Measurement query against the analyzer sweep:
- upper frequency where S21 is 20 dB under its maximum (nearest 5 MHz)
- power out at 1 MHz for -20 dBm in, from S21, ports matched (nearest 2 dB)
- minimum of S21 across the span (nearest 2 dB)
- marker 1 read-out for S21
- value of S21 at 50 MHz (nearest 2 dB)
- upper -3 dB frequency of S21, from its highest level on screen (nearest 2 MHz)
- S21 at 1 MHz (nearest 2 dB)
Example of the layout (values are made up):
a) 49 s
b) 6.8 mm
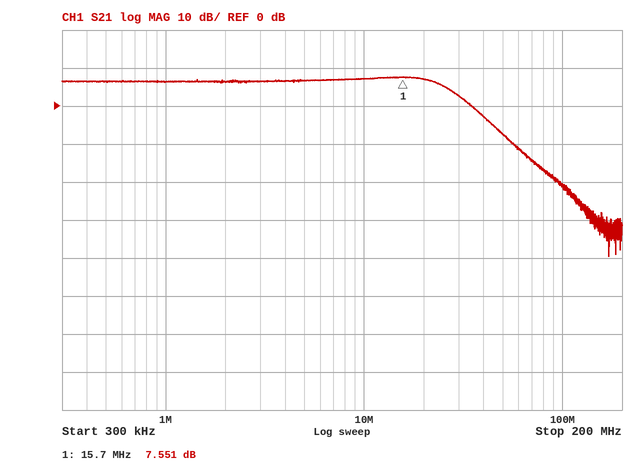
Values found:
a) 65 MHz
b) -14 dBm
c) -40 dB
d) 7.551 dB
e) -8 dB
f) 26 MHz
g) 6 dB
